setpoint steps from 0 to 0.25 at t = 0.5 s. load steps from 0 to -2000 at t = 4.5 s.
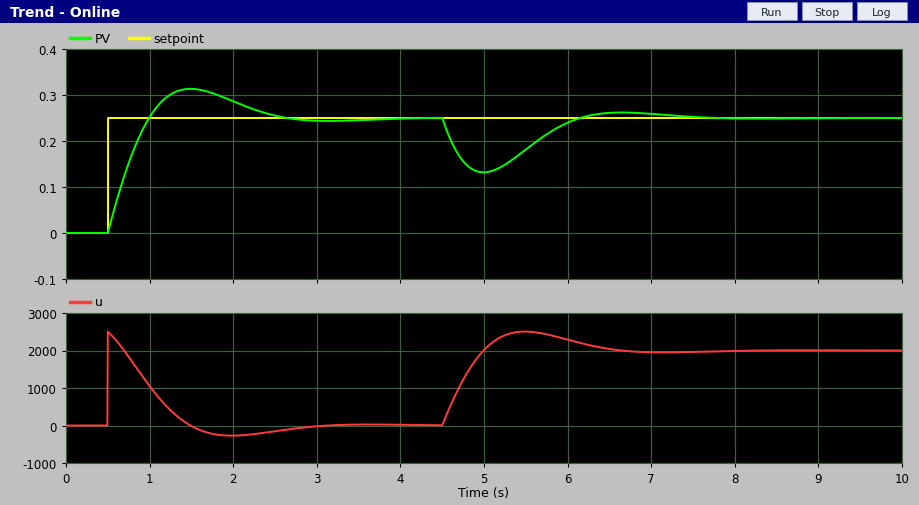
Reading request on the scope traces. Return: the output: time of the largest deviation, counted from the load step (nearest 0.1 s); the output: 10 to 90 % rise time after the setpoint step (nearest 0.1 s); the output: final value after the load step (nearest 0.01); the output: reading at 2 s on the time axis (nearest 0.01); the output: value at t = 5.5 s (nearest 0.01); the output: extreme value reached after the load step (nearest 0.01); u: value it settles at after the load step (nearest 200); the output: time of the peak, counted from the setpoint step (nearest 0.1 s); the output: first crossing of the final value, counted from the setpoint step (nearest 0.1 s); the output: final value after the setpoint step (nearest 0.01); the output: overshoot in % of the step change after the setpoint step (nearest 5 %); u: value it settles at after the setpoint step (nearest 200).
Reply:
0.5 s
0.4 s
0.25
0.29
0.18
0.13
2000
1.0 s
0.5 s
0.25
25 %
0
